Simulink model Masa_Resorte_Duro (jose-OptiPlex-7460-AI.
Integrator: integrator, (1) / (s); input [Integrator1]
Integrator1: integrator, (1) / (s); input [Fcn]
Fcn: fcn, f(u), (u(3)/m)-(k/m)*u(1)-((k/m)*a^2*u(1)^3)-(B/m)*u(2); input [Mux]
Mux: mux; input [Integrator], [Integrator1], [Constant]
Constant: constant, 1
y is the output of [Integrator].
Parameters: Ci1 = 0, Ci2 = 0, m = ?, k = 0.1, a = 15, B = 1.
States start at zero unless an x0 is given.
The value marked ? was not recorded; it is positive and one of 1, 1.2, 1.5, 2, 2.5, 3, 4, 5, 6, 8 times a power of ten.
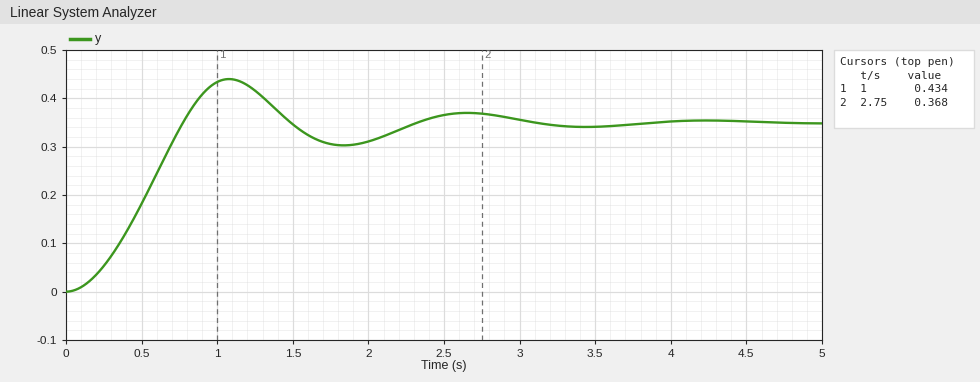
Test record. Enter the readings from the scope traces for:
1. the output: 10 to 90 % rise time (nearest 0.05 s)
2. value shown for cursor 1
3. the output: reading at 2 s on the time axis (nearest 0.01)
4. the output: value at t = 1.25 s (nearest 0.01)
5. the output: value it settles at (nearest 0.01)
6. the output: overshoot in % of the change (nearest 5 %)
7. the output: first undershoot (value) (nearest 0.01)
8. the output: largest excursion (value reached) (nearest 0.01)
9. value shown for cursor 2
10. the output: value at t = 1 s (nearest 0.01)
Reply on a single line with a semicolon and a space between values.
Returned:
0.50 s; 0.434; 0.31; 0.42; 0.35; 25 %; 0.30; 0.44; 0.368; 0.43
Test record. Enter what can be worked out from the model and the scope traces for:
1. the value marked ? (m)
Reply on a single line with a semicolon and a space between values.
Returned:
0.5
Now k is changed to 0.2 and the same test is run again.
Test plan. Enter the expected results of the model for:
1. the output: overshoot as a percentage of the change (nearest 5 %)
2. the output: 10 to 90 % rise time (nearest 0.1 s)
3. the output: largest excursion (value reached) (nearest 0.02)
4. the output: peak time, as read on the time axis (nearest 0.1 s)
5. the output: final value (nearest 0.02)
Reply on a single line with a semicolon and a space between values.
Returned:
30 %; 0.4 s; 0.36; 0.9 s; 0.28
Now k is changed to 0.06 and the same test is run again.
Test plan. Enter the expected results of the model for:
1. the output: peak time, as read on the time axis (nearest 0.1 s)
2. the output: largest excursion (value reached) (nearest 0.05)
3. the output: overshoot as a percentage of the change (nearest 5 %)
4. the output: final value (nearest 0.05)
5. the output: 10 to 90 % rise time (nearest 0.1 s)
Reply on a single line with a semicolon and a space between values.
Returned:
1.2 s; 0.50; 25 %; 0.40; 0.6 s
